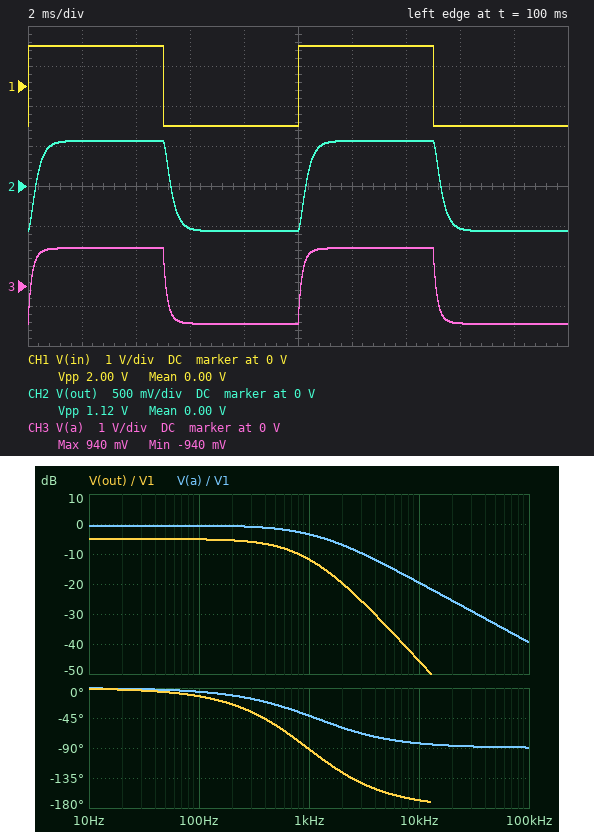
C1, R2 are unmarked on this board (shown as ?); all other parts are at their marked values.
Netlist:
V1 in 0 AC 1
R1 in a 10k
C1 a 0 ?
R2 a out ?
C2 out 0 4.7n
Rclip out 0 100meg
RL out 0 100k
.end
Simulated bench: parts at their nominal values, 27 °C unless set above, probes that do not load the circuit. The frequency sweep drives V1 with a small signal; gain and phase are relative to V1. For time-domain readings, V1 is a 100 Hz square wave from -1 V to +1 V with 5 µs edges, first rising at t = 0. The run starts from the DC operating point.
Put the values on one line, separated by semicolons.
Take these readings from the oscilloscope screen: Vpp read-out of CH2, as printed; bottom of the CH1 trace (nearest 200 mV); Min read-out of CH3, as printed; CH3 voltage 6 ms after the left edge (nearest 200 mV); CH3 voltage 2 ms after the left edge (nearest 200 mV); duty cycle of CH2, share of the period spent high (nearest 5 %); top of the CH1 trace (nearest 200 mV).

1.12 V; -1.0 V; -940 mV; -1.0 V; 1.0 V; 50 %; 1.0 V
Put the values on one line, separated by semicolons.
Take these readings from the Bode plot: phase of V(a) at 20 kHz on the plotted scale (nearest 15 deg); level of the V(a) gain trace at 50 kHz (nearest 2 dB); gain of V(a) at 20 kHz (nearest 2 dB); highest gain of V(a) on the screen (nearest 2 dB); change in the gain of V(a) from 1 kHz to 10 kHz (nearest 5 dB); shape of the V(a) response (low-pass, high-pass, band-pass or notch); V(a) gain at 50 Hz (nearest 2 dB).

-90 deg; -34 dB; -26 dB; 0 dB; -15 dB; low-pass; 0 dB
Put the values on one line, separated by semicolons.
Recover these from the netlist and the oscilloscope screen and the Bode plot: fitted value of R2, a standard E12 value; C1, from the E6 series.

68 kΩ; 15 nF
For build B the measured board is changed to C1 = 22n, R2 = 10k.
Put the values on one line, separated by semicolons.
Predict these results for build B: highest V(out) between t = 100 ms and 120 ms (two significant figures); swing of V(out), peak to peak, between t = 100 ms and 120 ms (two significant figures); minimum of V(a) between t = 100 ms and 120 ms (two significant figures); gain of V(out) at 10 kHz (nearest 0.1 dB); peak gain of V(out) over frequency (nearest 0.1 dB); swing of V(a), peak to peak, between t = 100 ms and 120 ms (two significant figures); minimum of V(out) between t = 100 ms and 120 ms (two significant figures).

830 mV; 1.7 V; -920 mV; -33.0 dB; -1.6 dB; 1.8 V; -830 mV
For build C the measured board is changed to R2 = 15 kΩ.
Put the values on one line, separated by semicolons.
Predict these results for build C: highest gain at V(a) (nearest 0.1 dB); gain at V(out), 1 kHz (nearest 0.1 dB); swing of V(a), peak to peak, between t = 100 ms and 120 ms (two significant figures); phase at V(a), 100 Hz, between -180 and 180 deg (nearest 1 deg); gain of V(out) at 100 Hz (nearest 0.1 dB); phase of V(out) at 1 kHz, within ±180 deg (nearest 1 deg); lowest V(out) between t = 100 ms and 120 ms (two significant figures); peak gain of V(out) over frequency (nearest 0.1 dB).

-0.7 dB; -6.0 dB; 1.8 V; -6 deg; -2.0 dB; -65 deg; -800 mV; -1.9 dB
